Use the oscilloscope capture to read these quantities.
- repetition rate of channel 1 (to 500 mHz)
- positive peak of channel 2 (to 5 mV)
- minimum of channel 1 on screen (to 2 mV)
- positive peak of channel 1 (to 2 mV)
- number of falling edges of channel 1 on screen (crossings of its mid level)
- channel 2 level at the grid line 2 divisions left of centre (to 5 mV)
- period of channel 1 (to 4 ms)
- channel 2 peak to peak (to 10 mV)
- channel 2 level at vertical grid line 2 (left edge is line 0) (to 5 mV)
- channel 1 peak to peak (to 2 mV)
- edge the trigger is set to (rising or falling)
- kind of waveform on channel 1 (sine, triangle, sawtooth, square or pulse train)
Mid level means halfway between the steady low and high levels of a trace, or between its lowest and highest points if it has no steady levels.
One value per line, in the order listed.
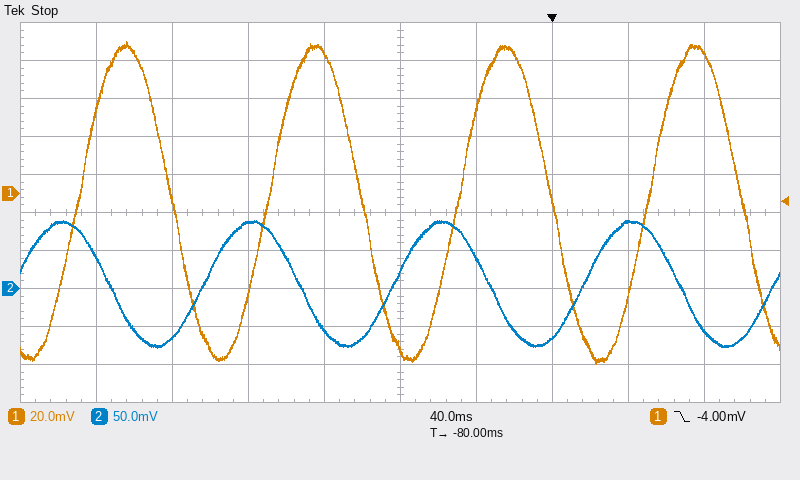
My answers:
10.0 Hz
90 mV
-90 mV
80 mV
4
85 mV
100 ms
170 mV
-65 mV
170 mV
falling
sine
